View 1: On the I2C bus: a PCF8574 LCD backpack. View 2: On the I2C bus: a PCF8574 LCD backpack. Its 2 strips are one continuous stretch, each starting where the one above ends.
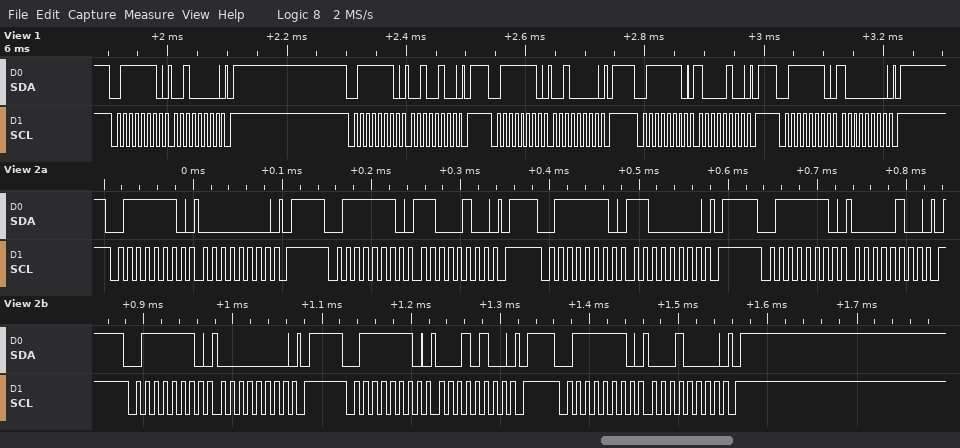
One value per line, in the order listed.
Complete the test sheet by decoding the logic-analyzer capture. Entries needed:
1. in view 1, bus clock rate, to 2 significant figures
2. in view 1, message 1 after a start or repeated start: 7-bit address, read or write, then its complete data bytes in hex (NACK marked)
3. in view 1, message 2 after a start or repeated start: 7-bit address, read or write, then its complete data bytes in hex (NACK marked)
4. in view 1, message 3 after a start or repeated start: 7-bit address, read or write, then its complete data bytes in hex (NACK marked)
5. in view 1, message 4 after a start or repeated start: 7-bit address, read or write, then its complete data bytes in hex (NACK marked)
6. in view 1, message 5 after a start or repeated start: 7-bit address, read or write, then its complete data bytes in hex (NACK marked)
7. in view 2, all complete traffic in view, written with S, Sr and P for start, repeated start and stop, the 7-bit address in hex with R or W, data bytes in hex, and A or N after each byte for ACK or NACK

100 kHz
0x3F write: 20
0x3F write: 24
0x3F write: 20
0x3F write: 84
0x3F write: 80
S 3FW A 00 A P S 3FW A C4 A P S 3FW A C0 A P S 3FW A 04 A P S 3FW A 00 A P S 3FW A 14 A P S 3FW A 10 A P
